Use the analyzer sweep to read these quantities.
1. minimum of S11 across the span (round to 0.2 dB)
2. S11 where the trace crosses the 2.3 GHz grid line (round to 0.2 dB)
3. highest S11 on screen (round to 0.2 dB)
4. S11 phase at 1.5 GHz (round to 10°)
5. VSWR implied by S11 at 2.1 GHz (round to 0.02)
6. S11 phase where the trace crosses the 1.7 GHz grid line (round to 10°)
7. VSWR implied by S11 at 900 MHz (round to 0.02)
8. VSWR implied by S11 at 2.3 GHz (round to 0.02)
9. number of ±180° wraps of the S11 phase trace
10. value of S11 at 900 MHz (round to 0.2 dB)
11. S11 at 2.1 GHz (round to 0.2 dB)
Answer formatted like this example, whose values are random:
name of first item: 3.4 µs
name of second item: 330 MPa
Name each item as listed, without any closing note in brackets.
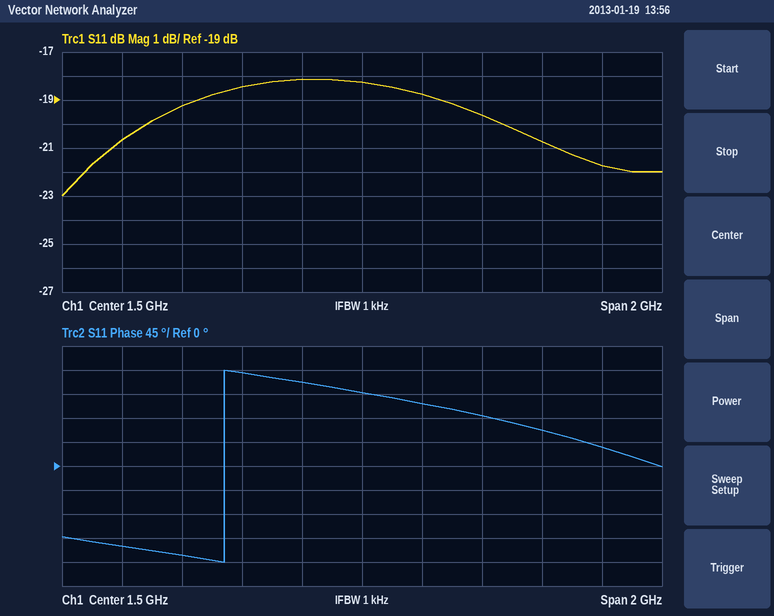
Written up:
minimum of S11 across the span: -23.0 dB
S11 where the trace crosses the 2.3 GHz grid line: -21.8 dB
highest S11 on screen: -18.2 dB
S11 phase at 1.5 GHz: 140°
VSWR implied by S11 at 2.1 GHz: 1.20
S11 phase where the trace crosses the 1.7 GHz grid line: 120°
VSWR implied by S11 at 900 MHz: 1.24
VSWR implied by S11 at 2.3 GHz: 1.18
number of ±180° wraps of the S11 phase trace: 1
value of S11 at 900 MHz: -19.2 dB
S11 at 2.1 GHz: -20.8 dB
